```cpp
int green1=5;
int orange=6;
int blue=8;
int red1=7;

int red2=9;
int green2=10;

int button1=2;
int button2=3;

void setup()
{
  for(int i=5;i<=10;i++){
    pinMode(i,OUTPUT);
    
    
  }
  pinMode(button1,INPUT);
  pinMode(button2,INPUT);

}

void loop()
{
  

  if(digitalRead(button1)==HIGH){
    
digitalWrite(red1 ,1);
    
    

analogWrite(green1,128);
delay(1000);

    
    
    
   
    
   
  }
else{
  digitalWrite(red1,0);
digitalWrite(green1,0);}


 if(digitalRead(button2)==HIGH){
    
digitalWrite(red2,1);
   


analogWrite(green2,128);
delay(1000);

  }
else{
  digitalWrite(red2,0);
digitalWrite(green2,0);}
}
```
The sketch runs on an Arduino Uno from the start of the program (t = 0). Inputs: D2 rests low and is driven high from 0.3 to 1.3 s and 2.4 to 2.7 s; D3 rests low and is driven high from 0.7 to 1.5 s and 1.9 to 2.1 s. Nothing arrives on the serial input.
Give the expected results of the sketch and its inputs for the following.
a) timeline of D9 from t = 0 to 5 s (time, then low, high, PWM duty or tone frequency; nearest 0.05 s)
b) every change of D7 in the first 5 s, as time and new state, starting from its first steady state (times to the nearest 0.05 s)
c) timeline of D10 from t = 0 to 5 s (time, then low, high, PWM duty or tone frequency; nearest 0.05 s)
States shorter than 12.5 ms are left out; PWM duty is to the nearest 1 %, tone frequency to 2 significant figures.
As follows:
0 s low; 1.3 s high; 2.3 s low
0 s low; 0.3 s high; 2.3 s low; 2.4 s high; 3.4 s low
0 s low; 1.3 s PWM 50 %; 2.3 s low
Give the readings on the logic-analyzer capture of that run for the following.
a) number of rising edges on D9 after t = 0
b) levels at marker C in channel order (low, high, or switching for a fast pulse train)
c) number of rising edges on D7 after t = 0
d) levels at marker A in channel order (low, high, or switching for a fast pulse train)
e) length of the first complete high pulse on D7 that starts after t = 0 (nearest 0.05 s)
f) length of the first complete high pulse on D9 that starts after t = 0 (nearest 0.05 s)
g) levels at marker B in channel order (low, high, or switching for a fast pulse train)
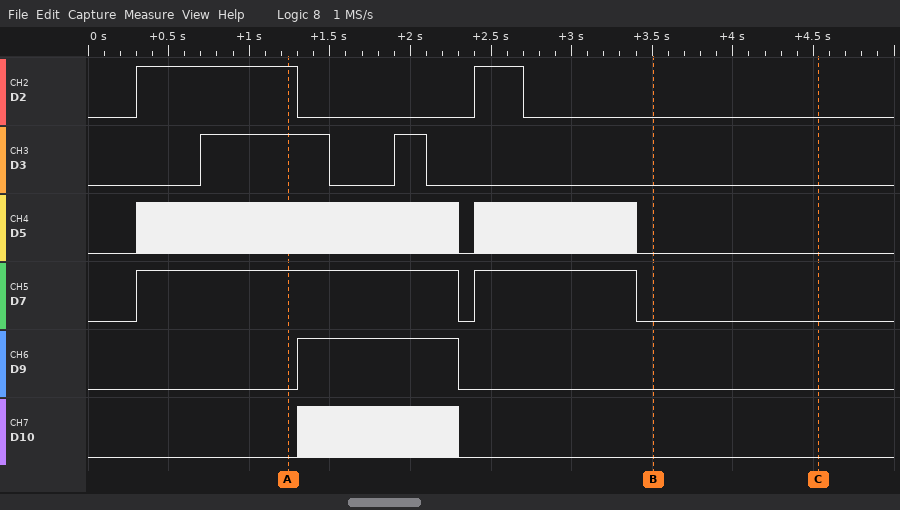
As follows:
1
D2 low, D3 low, D5 low, D7 low, D9 low, D10 low
2
D2 high, D3 high, D5 switching, D7 high, D9 low, D10 low
2.00 s
1.00 s
D2 low, D3 low, D5 low, D7 low, D9 low, D10 low
